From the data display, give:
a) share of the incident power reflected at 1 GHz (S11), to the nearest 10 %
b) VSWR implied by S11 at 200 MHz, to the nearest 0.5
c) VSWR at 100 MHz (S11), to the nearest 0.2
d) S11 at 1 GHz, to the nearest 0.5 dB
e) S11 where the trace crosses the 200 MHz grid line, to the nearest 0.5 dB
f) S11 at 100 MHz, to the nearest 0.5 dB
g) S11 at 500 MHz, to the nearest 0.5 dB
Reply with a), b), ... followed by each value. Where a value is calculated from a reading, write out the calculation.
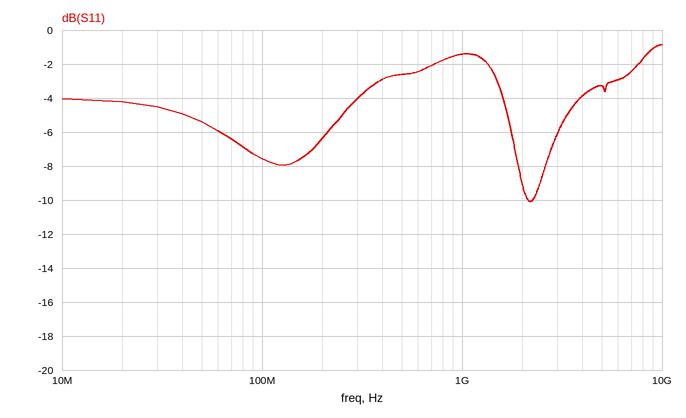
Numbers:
a) 10^(-1.5/10) ≈ 70.8 %, so 70 % to the nearest 10 %
b) |Γ| = 10^(-6.5/20) = 0.4732; VSWR = (1 + 0.4732)/(1 − 0.4732) ≈ 2.80, so 3.0 to the nearest 0.5
c) |Γ| = 10^(-7.5/20) = 0.4217; VSWR = (1 + 0.4217)/(1 − 0.4217) ≈ 2.46, so 2.4 to the nearest 0.2
d) -1.5 dB
e) -6.5 dB
f) -7.5 dB
g) -2.5 dB
